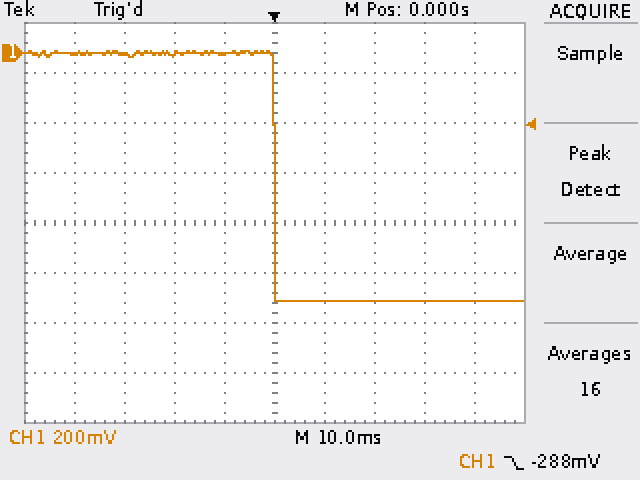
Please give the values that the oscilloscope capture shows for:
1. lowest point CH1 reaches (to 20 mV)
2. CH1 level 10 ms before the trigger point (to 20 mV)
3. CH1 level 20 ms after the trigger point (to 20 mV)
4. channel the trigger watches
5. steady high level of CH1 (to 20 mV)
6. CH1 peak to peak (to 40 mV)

-1.00 V
0 mV
-1.00 V
CH1
0 mV
1.00 V
